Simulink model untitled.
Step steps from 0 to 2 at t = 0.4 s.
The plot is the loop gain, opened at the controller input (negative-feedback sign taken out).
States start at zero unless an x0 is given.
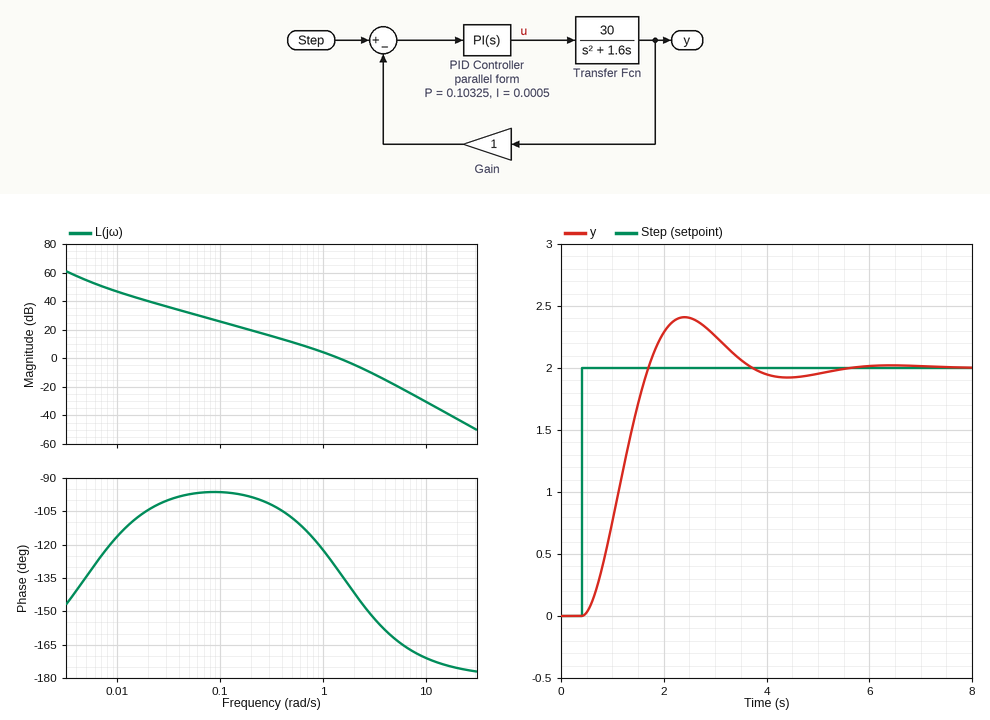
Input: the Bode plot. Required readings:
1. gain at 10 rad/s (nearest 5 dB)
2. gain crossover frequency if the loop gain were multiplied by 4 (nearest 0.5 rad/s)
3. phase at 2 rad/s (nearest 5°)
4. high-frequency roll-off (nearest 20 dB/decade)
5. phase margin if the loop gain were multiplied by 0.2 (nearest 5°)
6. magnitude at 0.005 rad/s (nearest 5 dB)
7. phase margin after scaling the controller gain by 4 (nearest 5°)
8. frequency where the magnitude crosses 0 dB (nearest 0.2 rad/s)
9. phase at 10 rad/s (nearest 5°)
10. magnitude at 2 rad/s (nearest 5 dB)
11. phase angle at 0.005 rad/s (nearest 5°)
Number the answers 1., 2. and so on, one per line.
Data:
1. -30 dB
2. 3.5 rad/s
3. -140°
4. -40 dB/decade
5. 75°
6. 55 dB
7. 25°
8. 1.4 rad/s
9. -170°
10. -5 dB
11. -135°
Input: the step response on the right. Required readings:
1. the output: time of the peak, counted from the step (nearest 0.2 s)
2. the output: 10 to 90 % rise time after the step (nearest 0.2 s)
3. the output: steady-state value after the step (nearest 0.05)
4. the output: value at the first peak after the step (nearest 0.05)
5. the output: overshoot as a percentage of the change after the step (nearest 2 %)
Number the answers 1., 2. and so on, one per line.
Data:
1. 2.0 s
2. 0.8 s
3. 2.00
4. 2.40
5. 20 %
